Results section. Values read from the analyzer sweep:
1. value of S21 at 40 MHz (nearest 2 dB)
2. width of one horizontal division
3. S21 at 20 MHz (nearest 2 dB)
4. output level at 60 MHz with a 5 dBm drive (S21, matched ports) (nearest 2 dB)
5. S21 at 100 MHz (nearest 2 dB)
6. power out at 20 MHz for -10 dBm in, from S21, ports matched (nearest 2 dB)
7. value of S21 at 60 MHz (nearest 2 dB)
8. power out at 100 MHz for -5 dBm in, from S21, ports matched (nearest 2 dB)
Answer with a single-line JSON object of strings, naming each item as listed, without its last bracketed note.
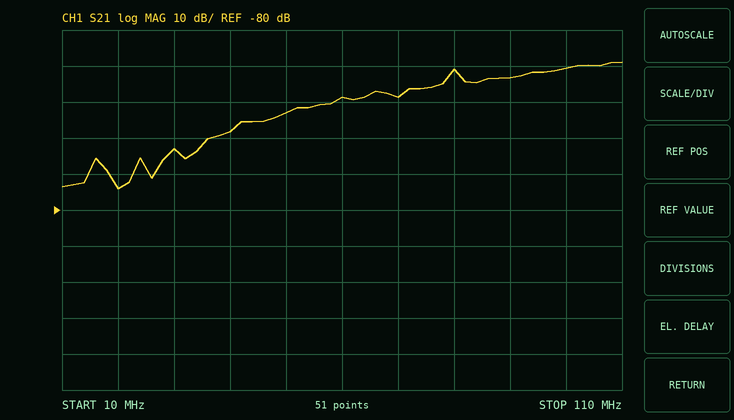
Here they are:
{"value of S21 at 40 MHz": "-58 dB", "width of one horizontal division": "10 MHz", "S21 at 20 MHz": "-74 dB", "output level at 60 MHz with a 5 dBm drive (S21, matched ports)": "-44 dBm", "S21 at 100 MHz": "-40 dB", "power out at 20 MHz for -10 dBm in, from S21, ports matched": "-84 dBm", "value of S21 at 60 MHz": "-48 dB", "power out at 100 MHz for -5 dBm in, from S21, ports matched": "-46 dBm"}
